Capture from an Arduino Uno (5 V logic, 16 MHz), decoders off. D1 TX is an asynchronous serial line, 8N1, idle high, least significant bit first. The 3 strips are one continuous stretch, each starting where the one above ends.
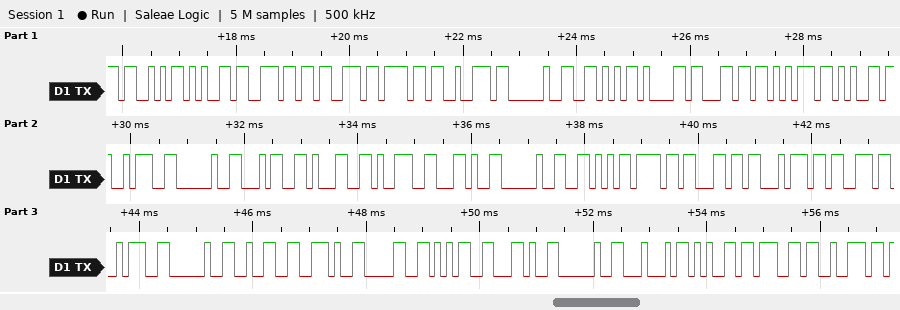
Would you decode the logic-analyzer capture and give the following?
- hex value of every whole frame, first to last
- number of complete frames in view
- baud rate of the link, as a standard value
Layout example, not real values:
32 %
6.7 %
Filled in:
53 65 6E 73 6F 72 20 56 61 6C 75 65 3A 20 34 31 39 2C 20 56 6F 6C 74 73 3A 20 32 2E 30 35 2C 20 44 65 67 72
36
9600 baud
